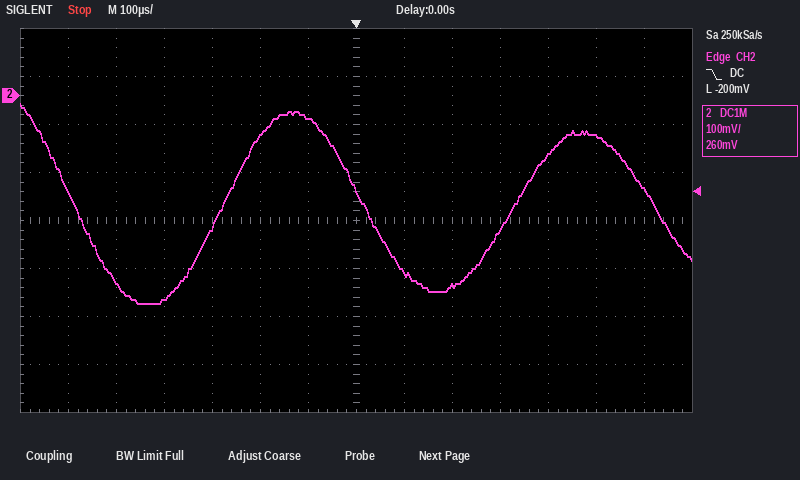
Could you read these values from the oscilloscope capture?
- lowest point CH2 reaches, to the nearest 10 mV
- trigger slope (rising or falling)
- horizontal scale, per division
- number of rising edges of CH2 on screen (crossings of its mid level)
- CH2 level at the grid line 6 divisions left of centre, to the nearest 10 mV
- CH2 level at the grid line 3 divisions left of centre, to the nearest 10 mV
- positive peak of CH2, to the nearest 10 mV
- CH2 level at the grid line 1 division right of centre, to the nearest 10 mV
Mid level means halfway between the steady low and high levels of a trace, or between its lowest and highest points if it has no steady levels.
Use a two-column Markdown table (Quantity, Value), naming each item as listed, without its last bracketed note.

| Quantity | Value |
|---|---|
| lowest point CH2 reaches, to the nearest 10 mV | -430 mV |
| trigger slope | falling |
| horizontal scale, per division | 100 µs |
| number of rising edges of CH2 on screen | 2 |
| CH2 level at the grid line 6 divisions left of centre, to the nearest 10 mV | -200 mV |
| CH2 level at the grid line 3 divisions left of centre, to the nearest 10 mV | -270 mV |
| positive peak of CH2, to the nearest 10 mV | -20 mV |
| CH2 level at the grid line 1 division right of centre, to the nearest 10 mV | -370 mV |
